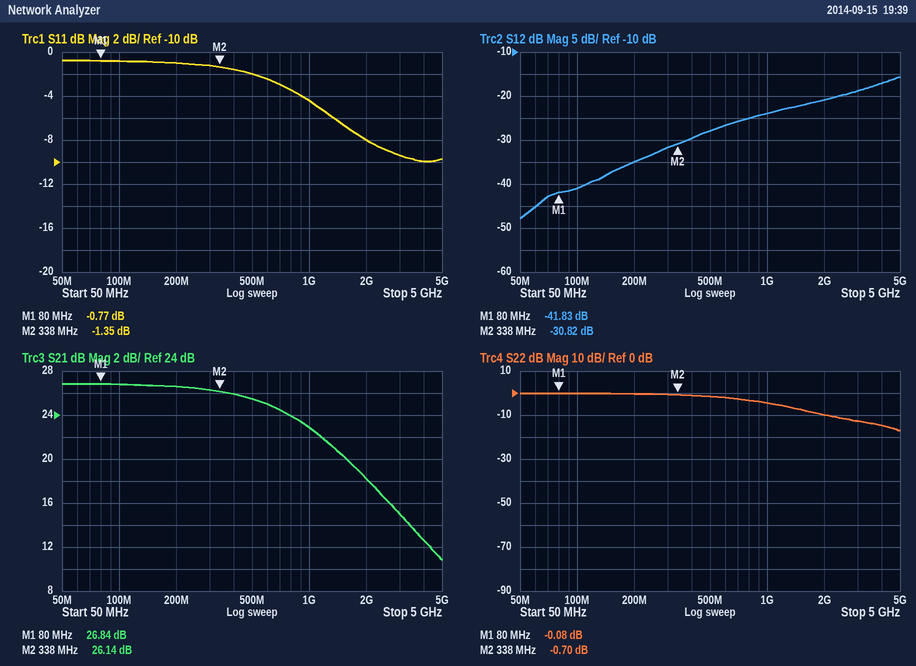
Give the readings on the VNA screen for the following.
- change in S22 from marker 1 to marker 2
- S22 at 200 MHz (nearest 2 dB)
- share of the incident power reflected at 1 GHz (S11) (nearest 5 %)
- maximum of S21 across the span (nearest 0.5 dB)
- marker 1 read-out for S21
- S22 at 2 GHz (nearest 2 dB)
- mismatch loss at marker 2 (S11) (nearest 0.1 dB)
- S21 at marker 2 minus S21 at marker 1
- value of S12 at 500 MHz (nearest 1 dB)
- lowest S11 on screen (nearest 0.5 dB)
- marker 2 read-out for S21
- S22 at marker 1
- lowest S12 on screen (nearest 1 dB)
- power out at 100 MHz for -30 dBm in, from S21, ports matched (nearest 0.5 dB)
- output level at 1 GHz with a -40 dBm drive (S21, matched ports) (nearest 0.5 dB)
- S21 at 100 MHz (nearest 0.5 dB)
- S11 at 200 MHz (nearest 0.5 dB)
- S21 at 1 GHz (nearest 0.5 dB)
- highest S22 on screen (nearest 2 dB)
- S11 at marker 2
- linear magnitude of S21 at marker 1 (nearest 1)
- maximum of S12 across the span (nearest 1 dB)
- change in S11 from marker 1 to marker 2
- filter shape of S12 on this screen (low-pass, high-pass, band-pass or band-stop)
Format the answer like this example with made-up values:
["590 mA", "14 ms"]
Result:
["-0.62 dB", "0 dB", "35 %", "27.0 dB", "26.84 dB", "-10 dB", "5.7 dB", "-0.70 dB", "-28 dB", "-10.0 dB", "26.14 dB", "-0.08 dB", "-48 dB", "-3.0 dBm", "-17.0 dBm", "27.0 dB", "-1.0 dB", "23.0 dB", "0 dB", "-1.35 dB", "22", "-16 dB", "-0.58 dB", "high-pass"]
